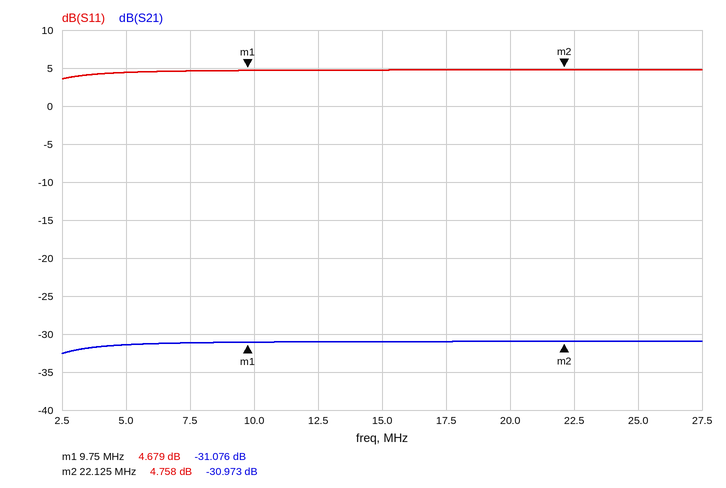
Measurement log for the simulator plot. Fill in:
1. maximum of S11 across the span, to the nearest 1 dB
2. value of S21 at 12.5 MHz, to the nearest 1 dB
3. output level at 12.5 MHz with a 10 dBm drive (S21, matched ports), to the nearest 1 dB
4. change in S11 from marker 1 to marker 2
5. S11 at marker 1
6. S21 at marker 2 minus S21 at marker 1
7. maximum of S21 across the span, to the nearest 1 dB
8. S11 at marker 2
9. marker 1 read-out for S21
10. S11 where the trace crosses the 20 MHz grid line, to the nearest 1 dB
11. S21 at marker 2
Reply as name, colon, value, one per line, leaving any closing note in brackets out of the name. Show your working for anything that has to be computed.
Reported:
maximum of S11 across the span, to the nearest 1 dB: 5 dB
value of S21 at 12.5 MHz, to the nearest 1 dB: -31 dB
output level at 12.5 MHz with a 10 dBm drive (S21, matched ports), to the nearest 1 dB: 10 dBm + (-31 dB) = -21 dBm
change in S11 from marker 1 to marker 2: 4.758 − (4.679) = 0.079 dB
S11 at marker 1: 4.679 dB
S21 at marker 2 minus S21 at marker 1: -30.973 − (-31.076) = 0.103 dB
maximum of S21 across the span, to the nearest 1 dB: -31 dB
S11 at marker 2: 4.758 dB
marker 1 read-out for S21: -31.076 dB
S11 where the trace crosses the 20 MHz grid line, to the nearest 1 dB: 5 dB
S21 at marker 2: -30.973 dB
